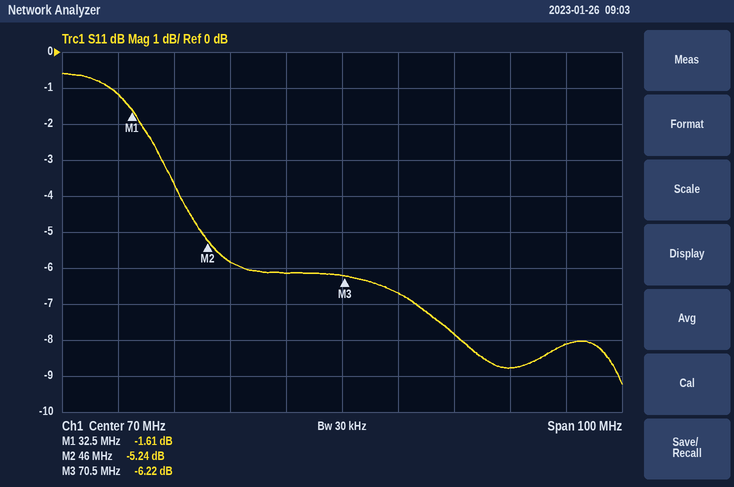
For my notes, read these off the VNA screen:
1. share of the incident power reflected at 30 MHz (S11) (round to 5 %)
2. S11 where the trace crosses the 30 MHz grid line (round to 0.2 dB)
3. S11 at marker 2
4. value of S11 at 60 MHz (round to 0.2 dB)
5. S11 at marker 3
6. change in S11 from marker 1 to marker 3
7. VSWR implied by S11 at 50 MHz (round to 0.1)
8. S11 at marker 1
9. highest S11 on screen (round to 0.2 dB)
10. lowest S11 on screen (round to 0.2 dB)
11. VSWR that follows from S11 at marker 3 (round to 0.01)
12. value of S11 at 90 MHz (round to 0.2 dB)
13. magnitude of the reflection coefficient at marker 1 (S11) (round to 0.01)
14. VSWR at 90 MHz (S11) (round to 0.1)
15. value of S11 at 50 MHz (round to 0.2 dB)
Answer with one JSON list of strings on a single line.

["75 %", "-1.2 dB", "-5.24 dB", "-6.2 dB", "-6.22 dB", "-4.61 dB", "3.1", "-1.61 dB", "-0.6 dB", "-9.2 dB", "2.91", "-7.8 dB", "0.83", "2.4", "-5.8 dB"]
